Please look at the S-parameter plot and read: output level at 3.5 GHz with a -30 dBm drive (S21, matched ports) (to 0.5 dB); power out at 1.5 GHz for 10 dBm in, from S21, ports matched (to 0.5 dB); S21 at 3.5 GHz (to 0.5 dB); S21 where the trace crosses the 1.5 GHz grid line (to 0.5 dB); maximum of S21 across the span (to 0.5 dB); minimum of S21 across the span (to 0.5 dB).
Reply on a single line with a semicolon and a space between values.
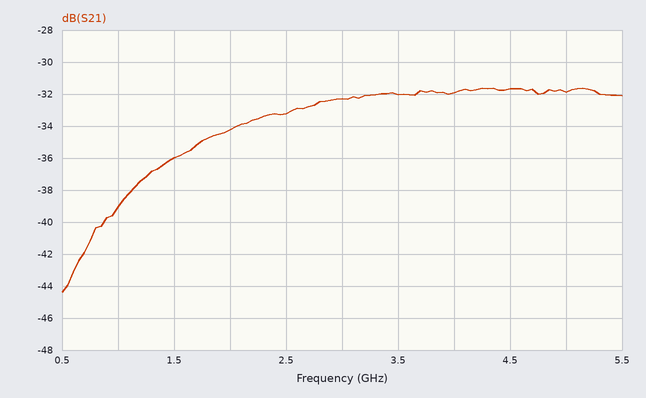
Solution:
-62.0 dBm; -26.0 dBm; -32.0 dB; -36.0 dB; -31.5 dB; -44.5 dB
